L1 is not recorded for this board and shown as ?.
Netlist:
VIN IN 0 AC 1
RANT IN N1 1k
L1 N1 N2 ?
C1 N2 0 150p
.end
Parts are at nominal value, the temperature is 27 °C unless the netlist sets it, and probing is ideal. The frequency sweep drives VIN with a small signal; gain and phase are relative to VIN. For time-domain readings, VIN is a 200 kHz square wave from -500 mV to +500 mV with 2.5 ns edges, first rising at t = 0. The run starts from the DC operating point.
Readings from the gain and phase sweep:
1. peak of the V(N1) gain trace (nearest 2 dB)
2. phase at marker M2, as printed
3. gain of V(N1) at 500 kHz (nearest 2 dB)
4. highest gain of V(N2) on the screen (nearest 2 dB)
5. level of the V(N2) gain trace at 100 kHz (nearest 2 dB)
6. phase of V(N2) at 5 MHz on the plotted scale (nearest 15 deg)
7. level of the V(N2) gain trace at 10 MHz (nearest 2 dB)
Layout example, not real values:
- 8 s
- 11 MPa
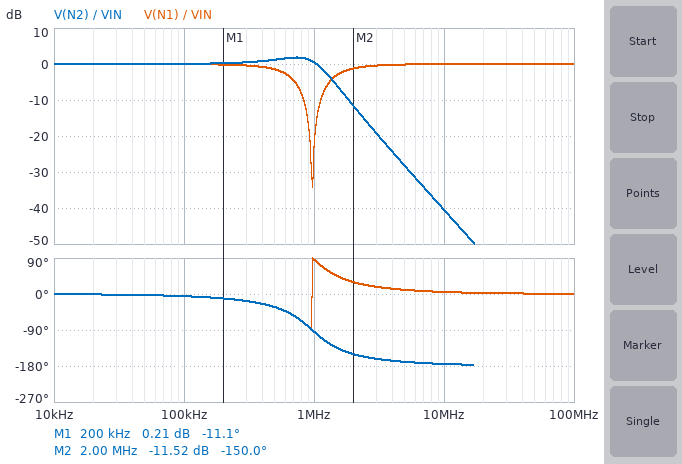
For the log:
- 0 dB
- -150.0 deg
- -2 dB
- 2 dB
- 0 dB
- -165 deg
- -40 dB
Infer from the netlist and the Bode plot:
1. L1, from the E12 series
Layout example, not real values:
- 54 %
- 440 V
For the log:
- 180 µH
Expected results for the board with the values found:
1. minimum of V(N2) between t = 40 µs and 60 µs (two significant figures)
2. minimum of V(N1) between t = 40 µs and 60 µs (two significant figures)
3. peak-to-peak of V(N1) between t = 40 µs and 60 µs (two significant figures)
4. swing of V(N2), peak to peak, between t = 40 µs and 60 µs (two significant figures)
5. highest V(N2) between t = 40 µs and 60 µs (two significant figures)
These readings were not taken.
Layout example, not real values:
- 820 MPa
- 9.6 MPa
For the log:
- -700 mV
- -600 mV
- 1.2 V
- 1.4 V
- 700 mV
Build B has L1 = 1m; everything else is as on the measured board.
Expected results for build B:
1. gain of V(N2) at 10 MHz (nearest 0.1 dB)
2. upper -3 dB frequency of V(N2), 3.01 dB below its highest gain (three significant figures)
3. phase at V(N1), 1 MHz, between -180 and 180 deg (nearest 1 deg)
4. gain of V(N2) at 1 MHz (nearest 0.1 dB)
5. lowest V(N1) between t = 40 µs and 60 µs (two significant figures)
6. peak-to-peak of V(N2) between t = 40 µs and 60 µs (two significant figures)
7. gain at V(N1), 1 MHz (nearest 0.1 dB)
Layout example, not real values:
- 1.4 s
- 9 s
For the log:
- -55.4 dB
- 469 kHz
- 11 deg
- -14.0 dB
- -620 mV
- 1.8 V
- -0.2 dB
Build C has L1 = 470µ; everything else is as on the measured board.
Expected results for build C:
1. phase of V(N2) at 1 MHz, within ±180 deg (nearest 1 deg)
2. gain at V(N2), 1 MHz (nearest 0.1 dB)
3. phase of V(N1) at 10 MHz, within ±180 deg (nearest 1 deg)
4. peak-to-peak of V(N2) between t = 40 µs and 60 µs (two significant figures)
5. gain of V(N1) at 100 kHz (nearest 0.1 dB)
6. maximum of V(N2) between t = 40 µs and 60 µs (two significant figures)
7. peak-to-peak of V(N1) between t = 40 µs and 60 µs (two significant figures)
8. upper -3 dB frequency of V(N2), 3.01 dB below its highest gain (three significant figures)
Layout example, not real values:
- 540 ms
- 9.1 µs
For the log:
- -152 deg
- -6.1 dB
- 2 deg
- 1.8 V
- 0 dB
- 920 mV
- 1.3 V
- 705 kHz
